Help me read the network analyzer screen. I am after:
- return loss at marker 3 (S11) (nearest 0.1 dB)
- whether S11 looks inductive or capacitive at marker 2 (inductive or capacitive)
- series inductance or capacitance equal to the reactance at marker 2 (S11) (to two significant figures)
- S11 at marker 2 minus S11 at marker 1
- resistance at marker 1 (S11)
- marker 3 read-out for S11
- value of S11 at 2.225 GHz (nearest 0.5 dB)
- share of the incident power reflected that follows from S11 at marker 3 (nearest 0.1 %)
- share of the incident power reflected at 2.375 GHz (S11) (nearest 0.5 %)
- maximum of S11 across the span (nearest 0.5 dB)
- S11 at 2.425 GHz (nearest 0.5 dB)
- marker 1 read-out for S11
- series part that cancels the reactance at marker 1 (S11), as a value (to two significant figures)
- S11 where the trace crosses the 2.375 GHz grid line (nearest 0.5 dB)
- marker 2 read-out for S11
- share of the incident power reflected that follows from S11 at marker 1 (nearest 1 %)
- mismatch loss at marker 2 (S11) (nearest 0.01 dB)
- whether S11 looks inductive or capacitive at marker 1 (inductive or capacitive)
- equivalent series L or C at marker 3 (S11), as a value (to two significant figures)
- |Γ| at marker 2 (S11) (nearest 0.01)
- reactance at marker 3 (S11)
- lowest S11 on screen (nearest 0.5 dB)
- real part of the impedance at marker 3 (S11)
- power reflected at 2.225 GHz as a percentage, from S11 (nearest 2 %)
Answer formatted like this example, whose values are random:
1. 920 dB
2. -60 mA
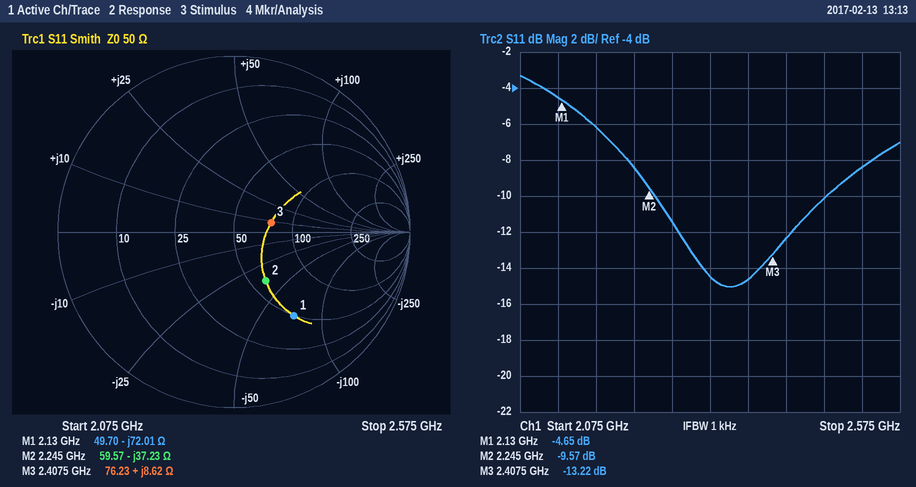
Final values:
1. 13.2 dB
2. capacitive
3. 1.9 pF
4. -4.92 dB
5. 49.70 Ω
6. -13.22 dB
7. -8.5 dB
8. 4.8 %
9. 3.5 %
10. -3.5 dB
11. -12.5 dB
12. -4.65 dB
13. 5.4 nH
14. -14.5 dB
15. -9.57 dB
16. 34 %
17. 0.51 dB
18. capacitive
19. 570 pH
20. 0.33
21. +8.62 Ω
22. -15.0 dB
23. 76.23 Ω
24. 14 %
